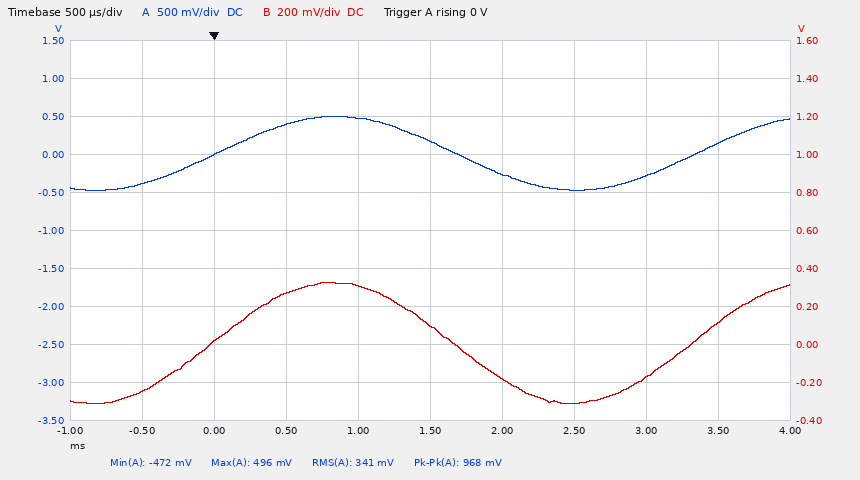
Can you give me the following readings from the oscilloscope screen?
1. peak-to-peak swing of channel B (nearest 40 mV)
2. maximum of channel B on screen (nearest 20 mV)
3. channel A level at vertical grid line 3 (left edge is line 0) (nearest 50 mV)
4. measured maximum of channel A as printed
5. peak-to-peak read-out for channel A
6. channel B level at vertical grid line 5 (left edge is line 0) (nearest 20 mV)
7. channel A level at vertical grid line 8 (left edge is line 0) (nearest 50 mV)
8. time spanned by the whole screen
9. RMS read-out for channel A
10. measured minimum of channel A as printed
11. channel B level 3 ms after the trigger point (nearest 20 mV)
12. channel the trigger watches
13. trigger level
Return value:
640 mV
320 mV
400 mV
496 mV
968 mV
100 mV
-300 mV
5 ms
341 mV
-472 mV
-180 mV
channel A
0 V
